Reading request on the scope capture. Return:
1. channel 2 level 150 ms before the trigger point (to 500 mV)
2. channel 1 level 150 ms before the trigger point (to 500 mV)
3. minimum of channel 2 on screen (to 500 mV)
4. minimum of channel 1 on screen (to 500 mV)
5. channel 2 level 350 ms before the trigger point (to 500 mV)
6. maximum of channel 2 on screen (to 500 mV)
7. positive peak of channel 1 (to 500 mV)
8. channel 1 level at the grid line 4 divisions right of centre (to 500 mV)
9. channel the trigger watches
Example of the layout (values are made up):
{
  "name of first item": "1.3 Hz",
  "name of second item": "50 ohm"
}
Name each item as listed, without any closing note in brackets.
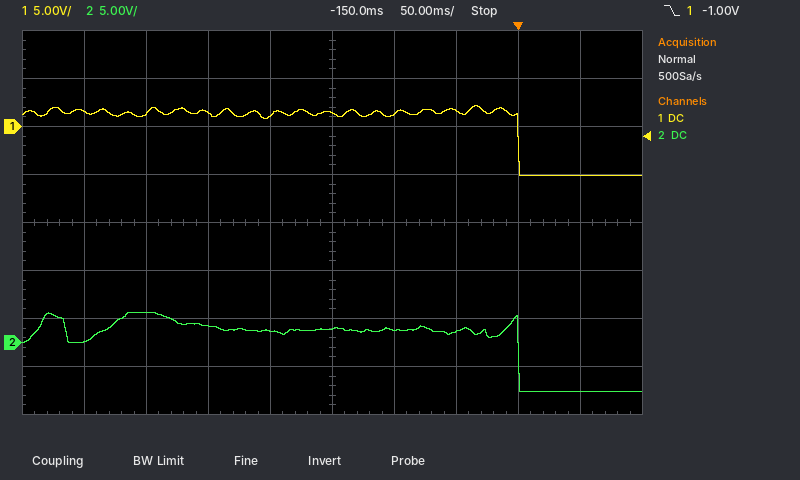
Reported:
{
  "channel 2 level 150 ms before the trigger point": "1.5 V",
  "channel 1 level 150 ms before the trigger point": "1.5 V",
  "minimum of channel 2 on screen": "-5.0 V",
  "minimum of channel 1 on screen": "-5.0 V",
  "channel 2 level 350 ms before the trigger point": "0.0 V",
  "maximum of channel 2 on screen": "3.0 V",
  "positive peak of channel 1": "2.0 V",
  "channel 1 level at the grid line 4 divisions right of centre": "-5.0 V",
  "channel the trigger watches": "channel 1"
}
